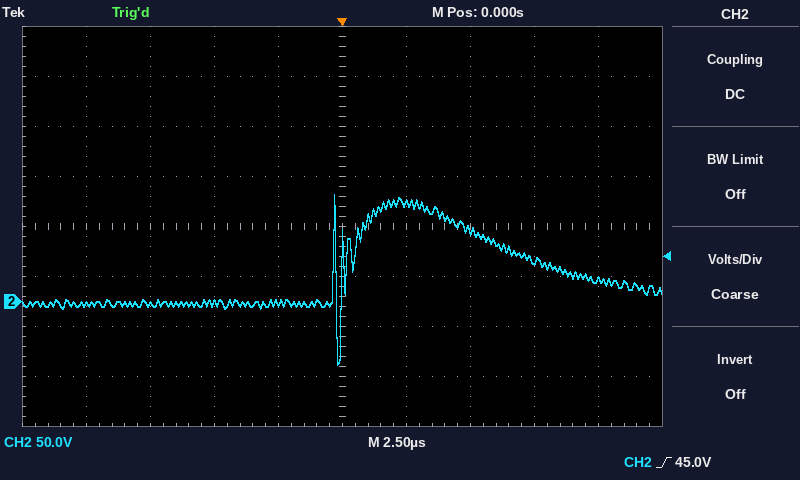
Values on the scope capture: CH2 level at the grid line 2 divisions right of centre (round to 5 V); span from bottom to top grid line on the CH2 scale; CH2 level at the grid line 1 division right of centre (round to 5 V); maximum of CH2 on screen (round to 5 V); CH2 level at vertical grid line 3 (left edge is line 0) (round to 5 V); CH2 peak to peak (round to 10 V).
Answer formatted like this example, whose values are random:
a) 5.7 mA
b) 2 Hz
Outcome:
a) 70 V
b) 400 V
c) 100 V
d) 105 V
e) 0 V
f) 170 V
